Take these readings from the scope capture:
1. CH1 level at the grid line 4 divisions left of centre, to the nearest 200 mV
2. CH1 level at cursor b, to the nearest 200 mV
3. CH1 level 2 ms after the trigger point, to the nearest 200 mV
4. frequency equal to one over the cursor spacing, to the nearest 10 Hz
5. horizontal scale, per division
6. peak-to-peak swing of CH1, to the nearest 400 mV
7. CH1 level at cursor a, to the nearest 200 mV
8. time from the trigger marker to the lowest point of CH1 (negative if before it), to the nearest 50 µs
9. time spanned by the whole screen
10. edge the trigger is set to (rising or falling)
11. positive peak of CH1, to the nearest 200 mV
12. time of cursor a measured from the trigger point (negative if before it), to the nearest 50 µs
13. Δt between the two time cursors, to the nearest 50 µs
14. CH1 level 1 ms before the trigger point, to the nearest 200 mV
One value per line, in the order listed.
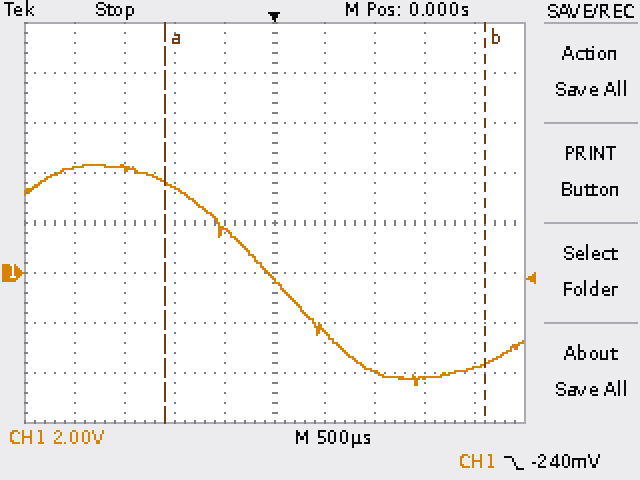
4.2 V
-3.6 V
-3.8 V
310 Hz
500 µs
8.8 V
3.6 V
+1.40 ms
5 ms
falling
4.4 V
-1.10 ms
3.20 ms
3.4 V
